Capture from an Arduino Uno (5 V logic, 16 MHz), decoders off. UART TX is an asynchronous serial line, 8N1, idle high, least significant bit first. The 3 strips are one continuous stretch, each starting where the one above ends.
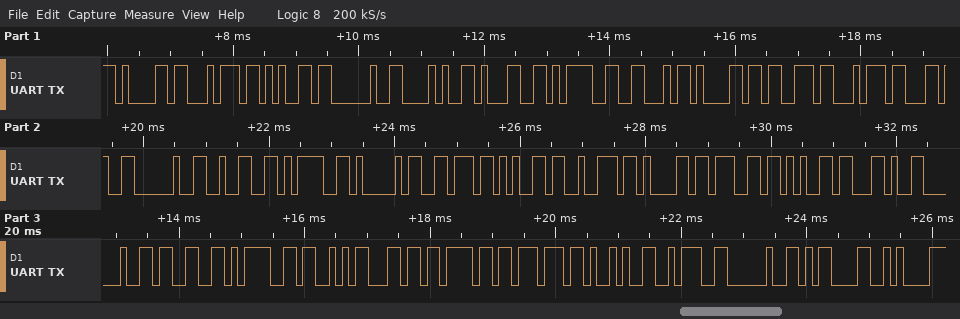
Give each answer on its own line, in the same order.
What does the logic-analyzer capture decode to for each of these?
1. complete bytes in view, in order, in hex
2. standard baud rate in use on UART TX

0x61 0x74 0x65 0x20 0x28 0x31 0x3D 0x46 0x61 0x73 0x74 0x2C 0x20 0x32 0x3D 0x41 0x76 0x65 0x72 0x61 0x67 0x65 0x2C 0x20 0x33 0x3D 0x53 0x6C 0x6F 0x77 0x29 0x3A 0x20 0x0D 0x0A
9600 baud
